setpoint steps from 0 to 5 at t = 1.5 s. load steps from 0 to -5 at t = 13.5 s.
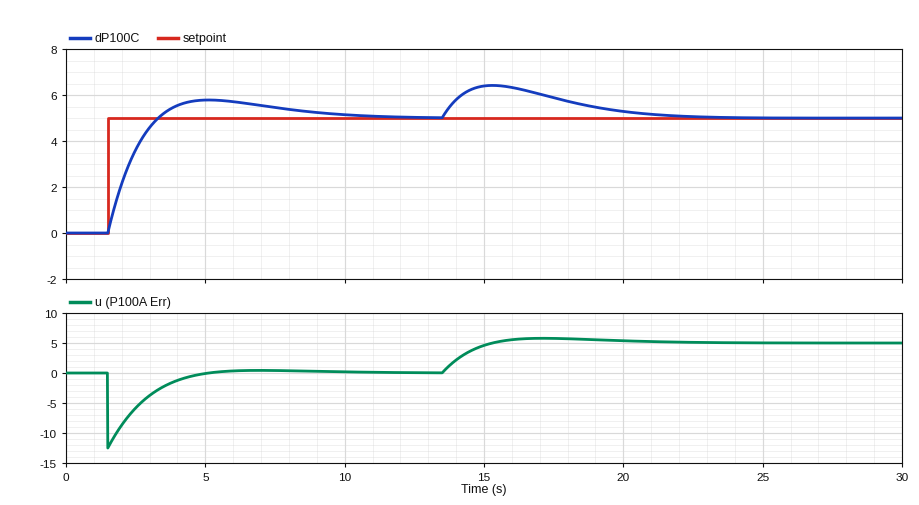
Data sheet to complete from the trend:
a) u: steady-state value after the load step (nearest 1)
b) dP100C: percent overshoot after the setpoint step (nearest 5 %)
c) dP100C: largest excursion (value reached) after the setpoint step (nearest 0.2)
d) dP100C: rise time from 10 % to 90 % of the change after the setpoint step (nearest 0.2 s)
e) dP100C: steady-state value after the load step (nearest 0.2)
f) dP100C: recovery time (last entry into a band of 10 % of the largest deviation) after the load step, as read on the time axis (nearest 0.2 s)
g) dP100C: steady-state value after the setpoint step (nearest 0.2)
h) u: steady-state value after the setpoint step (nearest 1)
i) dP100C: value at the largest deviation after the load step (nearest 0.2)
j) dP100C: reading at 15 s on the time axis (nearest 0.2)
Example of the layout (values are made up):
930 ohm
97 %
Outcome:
5
15 %
5.8
1.4 s
5.0
21.2 s
5.0
0
6.4
6.4
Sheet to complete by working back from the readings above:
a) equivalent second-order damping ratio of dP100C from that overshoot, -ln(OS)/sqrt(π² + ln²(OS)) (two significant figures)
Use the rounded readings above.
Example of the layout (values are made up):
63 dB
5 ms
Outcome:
0.52
